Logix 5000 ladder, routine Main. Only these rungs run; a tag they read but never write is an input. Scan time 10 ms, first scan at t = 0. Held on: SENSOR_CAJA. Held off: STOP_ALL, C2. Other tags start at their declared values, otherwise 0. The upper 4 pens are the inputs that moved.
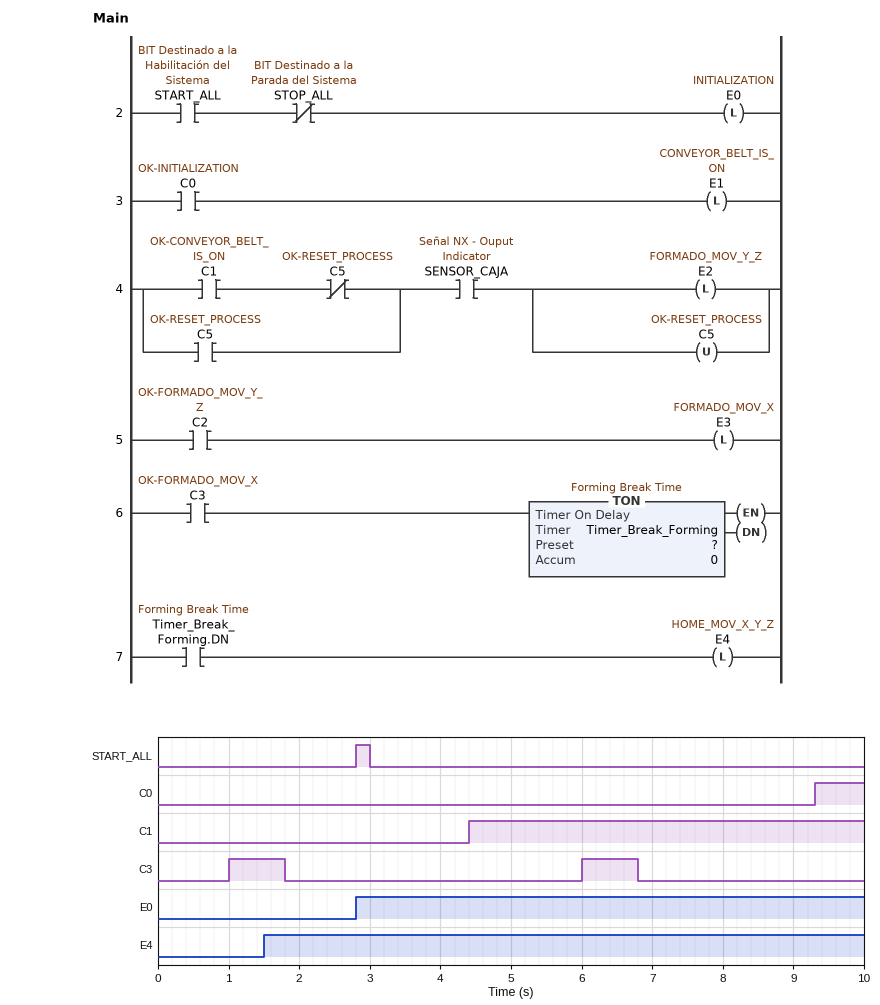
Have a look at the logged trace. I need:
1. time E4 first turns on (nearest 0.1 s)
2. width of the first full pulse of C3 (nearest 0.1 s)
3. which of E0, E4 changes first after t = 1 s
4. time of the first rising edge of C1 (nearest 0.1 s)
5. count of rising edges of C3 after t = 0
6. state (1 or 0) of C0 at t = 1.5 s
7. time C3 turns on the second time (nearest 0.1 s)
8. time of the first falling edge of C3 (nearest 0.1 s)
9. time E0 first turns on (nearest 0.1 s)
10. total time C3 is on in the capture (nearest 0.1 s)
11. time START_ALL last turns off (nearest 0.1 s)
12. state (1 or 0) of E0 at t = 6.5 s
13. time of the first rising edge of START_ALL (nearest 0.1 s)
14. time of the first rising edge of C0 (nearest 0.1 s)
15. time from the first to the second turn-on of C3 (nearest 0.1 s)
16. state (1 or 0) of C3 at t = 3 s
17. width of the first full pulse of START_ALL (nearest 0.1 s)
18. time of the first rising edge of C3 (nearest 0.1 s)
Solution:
1.5 s
0.8 s
E4
4.4 s
2
0
6.0 s
1.8 s
2.8 s
1.6 s
3.0 s
1
2.8 s
9.3 s
5.0 s
0
0.2 s
1.0 s
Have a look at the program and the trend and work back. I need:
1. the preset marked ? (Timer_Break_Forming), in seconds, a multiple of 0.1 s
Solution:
0.5 s
